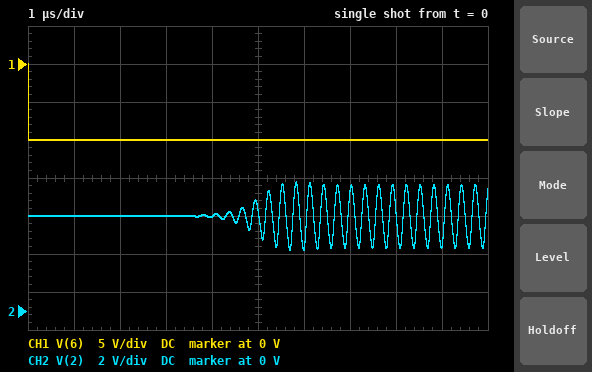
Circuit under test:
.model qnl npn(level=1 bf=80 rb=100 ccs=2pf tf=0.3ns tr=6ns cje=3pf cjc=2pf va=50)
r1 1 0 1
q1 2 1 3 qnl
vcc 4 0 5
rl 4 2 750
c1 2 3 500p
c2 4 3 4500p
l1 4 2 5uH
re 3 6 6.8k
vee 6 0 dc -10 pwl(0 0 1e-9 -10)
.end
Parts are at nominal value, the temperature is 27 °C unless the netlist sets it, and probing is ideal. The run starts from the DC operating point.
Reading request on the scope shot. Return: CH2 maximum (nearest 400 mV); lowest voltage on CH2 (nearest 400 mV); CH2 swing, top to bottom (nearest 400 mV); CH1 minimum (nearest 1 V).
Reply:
6.8 V
3.2 V
3.6 V
-10 V
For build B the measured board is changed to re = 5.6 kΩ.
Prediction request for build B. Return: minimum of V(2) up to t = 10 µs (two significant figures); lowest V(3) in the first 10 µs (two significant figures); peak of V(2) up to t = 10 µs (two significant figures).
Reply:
2.7 V
-860 mV
7.2 V
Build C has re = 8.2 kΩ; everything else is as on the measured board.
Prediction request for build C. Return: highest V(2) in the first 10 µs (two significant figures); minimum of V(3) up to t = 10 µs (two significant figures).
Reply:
6.4 V
-830 mV
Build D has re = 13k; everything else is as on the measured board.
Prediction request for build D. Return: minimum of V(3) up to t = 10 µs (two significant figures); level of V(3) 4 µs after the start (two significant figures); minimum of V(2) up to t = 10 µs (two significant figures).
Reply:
-760 mV
-600 mV
5.0 V
